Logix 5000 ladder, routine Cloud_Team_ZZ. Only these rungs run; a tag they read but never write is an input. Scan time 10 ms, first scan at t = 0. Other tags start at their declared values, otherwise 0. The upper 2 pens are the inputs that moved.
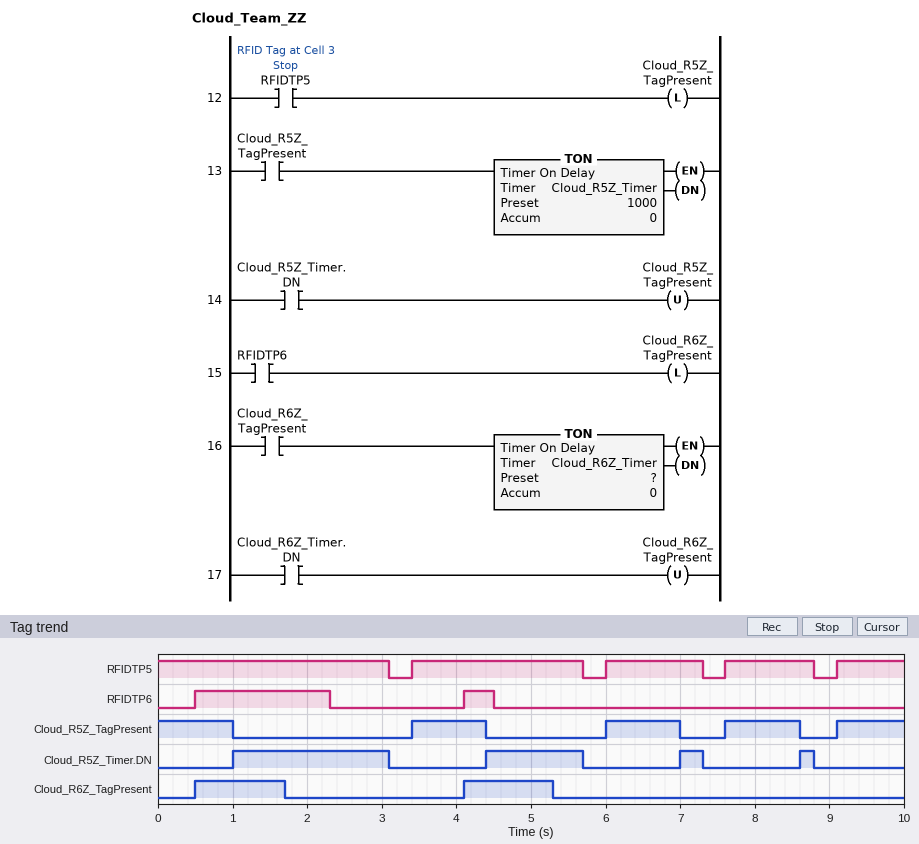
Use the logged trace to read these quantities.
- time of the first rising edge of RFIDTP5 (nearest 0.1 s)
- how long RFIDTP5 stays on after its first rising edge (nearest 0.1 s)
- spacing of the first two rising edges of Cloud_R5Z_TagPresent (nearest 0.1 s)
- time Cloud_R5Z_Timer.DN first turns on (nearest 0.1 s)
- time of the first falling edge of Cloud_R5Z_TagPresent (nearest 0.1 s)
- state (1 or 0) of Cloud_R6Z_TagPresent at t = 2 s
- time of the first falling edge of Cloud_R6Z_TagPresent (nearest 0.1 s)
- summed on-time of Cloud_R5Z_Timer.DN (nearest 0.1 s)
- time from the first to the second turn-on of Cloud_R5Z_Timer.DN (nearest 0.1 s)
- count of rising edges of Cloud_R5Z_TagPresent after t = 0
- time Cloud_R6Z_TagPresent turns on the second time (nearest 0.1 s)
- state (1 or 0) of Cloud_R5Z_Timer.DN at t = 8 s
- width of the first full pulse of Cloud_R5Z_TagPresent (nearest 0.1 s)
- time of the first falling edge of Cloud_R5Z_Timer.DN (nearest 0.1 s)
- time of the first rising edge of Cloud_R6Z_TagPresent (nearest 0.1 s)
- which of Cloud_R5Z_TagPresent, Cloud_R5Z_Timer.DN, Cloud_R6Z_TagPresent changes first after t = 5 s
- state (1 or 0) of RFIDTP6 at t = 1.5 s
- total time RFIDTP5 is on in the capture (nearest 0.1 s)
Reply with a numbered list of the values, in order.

1. 3.4 s
2. 2.3 s
3. 2.6 s
4. 1.0 s
5. 1.0 s
6. 0
7. 1.7 s
8. 3.9 s
9. 3.4 s
10. 4
11. 4.1 s
12. 0
13. 1.0 s
14. 3.1 s
15. 0.5 s
16. Cloud_R6Z_TagPresent
17. 1
18. 8.8 s
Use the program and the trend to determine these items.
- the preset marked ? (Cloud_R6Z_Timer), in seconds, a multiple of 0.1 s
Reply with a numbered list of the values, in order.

1. 1.2 s
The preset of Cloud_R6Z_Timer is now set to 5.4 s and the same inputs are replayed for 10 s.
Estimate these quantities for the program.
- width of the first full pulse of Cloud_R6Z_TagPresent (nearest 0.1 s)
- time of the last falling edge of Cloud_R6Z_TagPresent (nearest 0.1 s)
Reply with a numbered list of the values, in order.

1. 5.4 s
2. 5.9 s
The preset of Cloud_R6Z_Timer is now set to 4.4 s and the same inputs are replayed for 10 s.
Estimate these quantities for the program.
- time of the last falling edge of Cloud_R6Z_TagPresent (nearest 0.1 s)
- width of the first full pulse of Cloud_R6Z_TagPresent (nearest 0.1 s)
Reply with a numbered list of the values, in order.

1. 4.9 s
2. 4.4 s
